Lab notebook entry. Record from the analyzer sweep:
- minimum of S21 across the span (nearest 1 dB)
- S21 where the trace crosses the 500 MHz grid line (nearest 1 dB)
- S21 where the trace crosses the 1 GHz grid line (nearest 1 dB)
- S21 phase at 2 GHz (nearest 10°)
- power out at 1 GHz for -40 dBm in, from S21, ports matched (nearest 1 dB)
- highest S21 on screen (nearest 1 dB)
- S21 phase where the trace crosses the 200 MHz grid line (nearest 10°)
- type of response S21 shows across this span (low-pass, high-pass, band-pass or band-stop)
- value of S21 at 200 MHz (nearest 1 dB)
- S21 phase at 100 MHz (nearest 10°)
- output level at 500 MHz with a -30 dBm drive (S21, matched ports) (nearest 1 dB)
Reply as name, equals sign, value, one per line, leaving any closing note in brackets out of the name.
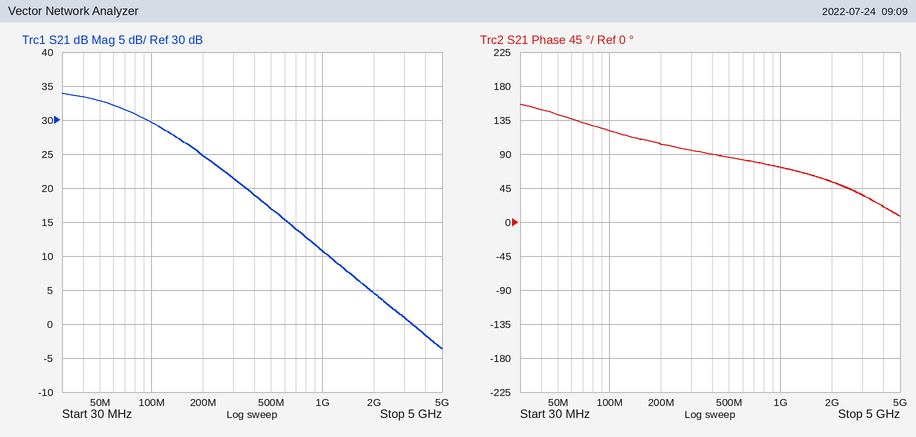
minimum of S21 across the span = -4 dB
S21 where the trace crosses the 500 MHz grid line = 17 dB
S21 where the trace crosses the 1 GHz grid line = 11 dB
S21 phase at 2 GHz = 50°
power out at 1 GHz for -40 dBm in, from S21, ports matched = -29 dBm
highest S21 on screen = 34 dB
S21 phase where the trace crosses the 200 MHz grid line = 100°
type of response S21 shows across this span = low-pass
value of S21 at 200 MHz = 25 dB
S21 phase at 100 MHz = 120°
output level at 500 MHz with a -30 dBm drive (S21, matched ports) = -13 dBm
